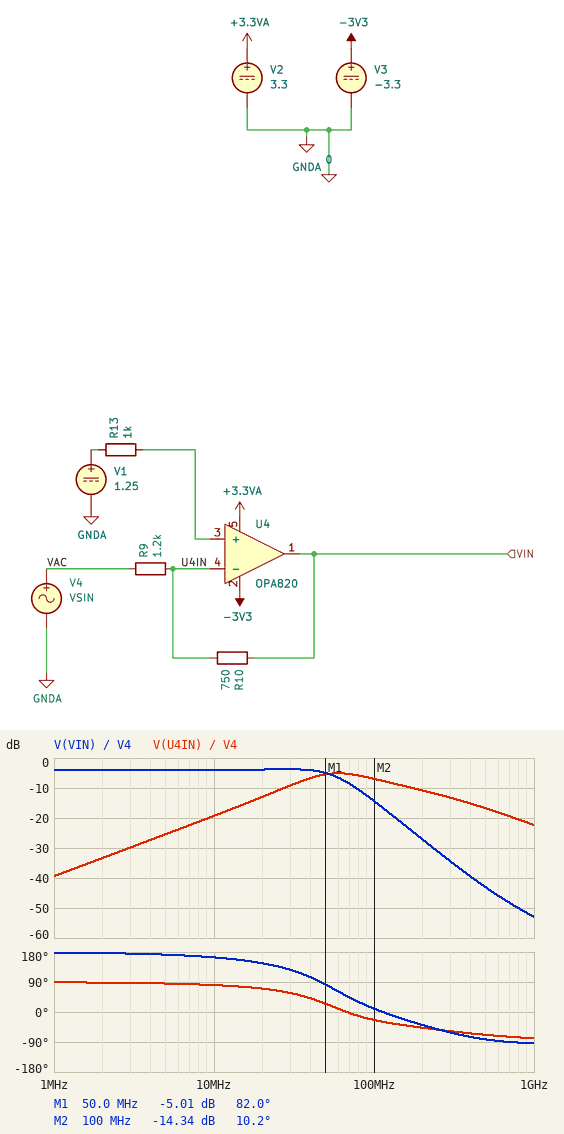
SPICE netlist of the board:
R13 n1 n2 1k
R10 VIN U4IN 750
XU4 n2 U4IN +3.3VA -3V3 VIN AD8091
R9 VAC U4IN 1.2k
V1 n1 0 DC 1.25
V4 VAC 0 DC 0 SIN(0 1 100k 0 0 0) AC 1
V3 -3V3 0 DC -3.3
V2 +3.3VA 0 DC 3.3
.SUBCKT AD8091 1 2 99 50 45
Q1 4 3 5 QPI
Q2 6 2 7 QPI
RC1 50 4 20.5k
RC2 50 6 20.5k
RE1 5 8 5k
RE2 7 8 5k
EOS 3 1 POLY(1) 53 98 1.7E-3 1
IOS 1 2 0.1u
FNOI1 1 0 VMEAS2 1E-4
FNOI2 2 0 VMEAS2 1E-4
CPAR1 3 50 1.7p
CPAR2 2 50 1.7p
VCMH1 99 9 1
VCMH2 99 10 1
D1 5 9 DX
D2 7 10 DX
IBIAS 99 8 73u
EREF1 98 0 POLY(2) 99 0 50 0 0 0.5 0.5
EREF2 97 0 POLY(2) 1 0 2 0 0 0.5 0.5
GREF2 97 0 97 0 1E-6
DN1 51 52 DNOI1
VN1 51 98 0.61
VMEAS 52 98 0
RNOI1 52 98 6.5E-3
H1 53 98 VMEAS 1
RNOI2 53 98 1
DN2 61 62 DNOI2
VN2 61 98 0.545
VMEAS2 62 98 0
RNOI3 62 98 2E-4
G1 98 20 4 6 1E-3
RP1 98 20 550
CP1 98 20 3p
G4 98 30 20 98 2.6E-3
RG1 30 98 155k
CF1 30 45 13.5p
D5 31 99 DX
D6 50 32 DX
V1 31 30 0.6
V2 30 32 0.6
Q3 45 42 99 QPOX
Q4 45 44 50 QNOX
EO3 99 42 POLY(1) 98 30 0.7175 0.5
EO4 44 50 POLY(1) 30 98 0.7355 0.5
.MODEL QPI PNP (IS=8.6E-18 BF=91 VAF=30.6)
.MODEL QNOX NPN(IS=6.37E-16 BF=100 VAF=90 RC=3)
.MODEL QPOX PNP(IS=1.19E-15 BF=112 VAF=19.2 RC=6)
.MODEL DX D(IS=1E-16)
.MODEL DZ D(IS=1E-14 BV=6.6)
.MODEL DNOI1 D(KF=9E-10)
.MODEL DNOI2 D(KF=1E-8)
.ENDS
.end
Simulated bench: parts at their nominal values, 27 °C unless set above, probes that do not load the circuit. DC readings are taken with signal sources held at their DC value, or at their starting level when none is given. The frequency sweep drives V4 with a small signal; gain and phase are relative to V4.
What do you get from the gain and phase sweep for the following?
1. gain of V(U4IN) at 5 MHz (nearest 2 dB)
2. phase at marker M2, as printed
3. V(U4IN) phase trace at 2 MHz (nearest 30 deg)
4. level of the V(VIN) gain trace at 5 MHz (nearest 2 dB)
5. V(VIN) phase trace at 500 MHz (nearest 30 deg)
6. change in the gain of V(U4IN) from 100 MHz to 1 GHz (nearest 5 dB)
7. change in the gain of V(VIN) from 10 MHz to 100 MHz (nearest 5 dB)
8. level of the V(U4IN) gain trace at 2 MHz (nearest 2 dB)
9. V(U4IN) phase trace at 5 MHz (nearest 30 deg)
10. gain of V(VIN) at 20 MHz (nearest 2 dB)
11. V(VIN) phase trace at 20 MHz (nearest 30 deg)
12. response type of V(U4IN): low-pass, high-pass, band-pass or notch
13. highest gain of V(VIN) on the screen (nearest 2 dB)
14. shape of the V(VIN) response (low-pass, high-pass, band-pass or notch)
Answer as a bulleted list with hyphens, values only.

- -26 dB
- 10.2 deg
- 90 deg
- -4 dB
- -90 deg
- -15 dB
- -10 dB
- -34 dB
- 90 deg
- -4 dB
- 150 deg
- band-pass
- -4 dB
- low-pass
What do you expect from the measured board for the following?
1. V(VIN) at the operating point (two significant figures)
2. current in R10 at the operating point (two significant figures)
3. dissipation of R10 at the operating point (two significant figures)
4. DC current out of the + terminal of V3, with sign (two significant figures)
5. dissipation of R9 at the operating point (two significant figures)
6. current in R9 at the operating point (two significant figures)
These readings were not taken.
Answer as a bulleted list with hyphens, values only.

- 2.0 V
- 1.0 mA
- 820 µW
- -1.1 mA
- 1.3 mW
- 1.0 mA
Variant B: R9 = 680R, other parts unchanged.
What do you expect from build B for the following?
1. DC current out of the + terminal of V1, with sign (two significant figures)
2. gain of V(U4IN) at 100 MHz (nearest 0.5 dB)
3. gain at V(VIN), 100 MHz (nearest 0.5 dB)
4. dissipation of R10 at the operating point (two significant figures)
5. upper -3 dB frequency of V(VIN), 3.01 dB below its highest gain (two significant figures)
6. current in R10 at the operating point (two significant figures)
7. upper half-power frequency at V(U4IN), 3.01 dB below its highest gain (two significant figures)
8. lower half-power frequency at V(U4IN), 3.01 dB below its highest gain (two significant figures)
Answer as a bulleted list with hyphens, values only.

- -250 nA
- -4.5 dB
- -12.0 dB
- 2.5 mW
- 45 MHz
- 1.8 mA
- 160 MHz
- 27 MHz
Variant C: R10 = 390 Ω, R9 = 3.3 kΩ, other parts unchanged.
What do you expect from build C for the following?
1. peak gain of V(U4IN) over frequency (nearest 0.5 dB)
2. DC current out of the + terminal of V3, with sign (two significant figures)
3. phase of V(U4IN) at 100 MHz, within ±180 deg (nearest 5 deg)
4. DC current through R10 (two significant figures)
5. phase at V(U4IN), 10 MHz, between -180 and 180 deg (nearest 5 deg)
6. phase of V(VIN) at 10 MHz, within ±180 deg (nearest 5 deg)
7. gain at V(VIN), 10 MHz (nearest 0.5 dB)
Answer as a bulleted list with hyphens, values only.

- -15.0 dB
- -1.3 mA
- -15 deg
- 380 µA
- 85 deg
- 170 deg
- -18.5 dB
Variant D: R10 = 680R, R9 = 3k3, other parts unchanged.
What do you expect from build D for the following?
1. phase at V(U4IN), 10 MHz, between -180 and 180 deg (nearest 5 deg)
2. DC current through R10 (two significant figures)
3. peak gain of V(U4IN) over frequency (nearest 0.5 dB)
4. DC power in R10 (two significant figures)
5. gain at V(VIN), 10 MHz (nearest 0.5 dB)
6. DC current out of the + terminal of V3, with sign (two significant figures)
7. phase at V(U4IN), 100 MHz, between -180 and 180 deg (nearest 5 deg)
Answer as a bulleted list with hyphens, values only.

- 85 deg
- 380 µA
- -11.0 dB
- 98 µW
- -13.5 dB
- -1.3 mA
- -30 deg
